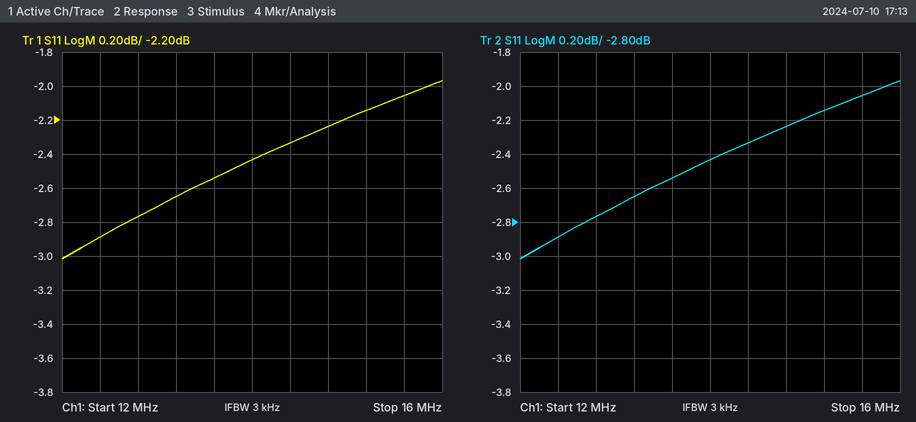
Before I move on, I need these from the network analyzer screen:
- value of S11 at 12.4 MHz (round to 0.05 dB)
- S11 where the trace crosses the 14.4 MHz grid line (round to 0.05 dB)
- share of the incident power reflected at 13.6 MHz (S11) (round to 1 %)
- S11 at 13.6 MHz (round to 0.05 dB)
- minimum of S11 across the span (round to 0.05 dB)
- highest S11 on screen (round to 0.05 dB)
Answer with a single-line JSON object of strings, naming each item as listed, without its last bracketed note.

{"value of S11 at 12.4 MHz": "-2.90 dB", "S11 where the trace crosses the 14.4 MHz grid line": "-2.35 dB", "share of the incident power reflected at 13.6 MHz (S11)": "56 %", "S11 at 13.6 MHz": "-2.55 dB", "minimum of S11 across the span": "-3.00 dB", "highest S11 on screen": "-1.95 dB"}
